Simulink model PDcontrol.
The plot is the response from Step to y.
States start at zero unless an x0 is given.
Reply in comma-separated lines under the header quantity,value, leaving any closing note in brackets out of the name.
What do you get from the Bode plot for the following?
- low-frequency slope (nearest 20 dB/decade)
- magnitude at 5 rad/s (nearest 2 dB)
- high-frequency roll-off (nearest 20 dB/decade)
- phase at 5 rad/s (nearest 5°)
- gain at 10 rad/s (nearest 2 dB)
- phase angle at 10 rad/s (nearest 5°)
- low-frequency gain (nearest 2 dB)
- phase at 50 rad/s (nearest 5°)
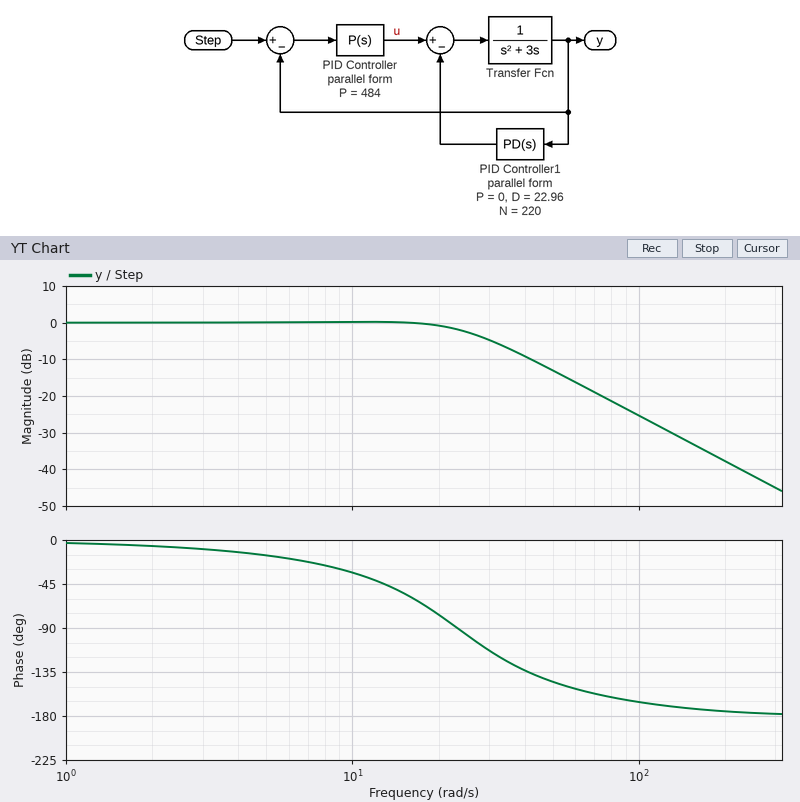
quantity,value
low-frequency slope,0 dB/decade
magnitude at 5 rad/s,0 dB
high-frequency roll-off,-40 dB/decade
phase at 5 rad/s,-15°
gain at 10 rad/s,0 dB
phase angle at 10 rad/s,-35°
low-frequency gain,0 dB
phase at 50 rad/s,-145°
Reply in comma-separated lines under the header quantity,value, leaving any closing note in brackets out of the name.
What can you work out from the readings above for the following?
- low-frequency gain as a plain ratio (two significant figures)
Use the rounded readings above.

quantity,value
low-frequency gain as a plain ratio,1.0
